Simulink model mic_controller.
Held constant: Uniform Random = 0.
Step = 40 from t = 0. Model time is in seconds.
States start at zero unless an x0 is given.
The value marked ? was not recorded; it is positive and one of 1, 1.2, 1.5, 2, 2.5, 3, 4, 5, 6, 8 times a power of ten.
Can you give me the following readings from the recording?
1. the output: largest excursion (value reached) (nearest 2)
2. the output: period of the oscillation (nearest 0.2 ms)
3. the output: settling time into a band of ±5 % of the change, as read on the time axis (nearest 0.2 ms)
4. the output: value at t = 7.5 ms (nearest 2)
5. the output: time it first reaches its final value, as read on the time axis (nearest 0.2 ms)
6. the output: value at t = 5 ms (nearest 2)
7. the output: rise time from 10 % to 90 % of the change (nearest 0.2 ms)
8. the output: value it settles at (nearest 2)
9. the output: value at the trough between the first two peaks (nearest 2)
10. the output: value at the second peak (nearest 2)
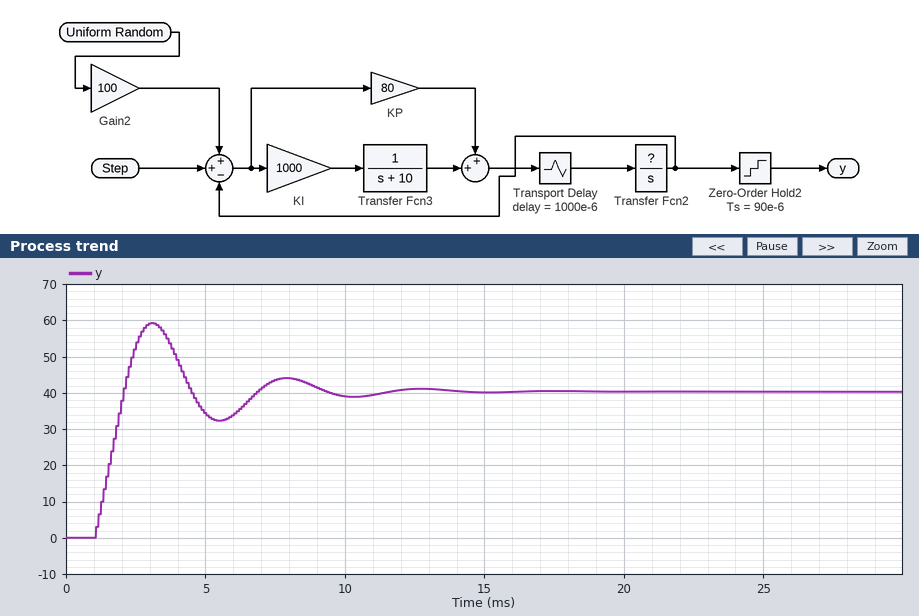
60
4.8 ms
8.8 ms
44
2.0 ms
34
0.8 ms
40
32
44
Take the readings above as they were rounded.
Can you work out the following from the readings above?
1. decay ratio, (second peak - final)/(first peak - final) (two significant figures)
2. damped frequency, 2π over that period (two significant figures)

0.20
1.3 rad/ms
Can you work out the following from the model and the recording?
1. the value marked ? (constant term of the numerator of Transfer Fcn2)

12
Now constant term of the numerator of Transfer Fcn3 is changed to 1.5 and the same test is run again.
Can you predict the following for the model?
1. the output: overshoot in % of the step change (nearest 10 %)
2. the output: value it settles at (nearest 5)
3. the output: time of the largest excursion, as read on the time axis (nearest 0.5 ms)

50 %
40
3.0 ms
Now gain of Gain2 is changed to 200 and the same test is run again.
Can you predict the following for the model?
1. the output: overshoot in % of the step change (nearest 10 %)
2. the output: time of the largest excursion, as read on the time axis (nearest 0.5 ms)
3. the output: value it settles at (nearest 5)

50 %
3.0 ms
40
